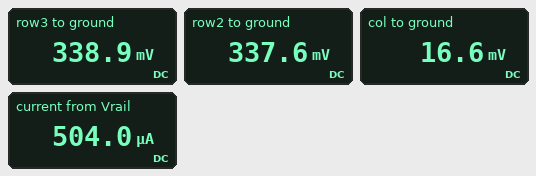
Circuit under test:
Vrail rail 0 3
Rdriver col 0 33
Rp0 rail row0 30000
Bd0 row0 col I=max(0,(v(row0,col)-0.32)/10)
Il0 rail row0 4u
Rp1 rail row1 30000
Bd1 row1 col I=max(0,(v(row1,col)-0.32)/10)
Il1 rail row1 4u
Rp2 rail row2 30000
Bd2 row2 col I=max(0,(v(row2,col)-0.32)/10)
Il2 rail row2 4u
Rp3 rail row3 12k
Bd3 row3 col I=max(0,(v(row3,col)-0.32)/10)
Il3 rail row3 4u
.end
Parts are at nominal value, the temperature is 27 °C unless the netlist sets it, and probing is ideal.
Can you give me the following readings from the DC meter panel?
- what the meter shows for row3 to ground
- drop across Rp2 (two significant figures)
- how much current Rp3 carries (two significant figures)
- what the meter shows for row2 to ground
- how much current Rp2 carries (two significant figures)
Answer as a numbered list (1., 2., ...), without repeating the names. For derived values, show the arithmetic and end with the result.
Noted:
1. 338.9 mV
2. 3 V - 337.6 mV = 2.7 V
3. (3 V - 338.9 mV) / 12 kΩ = 220 µA
4. 337.6 mV
5. (3 V - 337.6 mV) / 30 kΩ = 89 µA
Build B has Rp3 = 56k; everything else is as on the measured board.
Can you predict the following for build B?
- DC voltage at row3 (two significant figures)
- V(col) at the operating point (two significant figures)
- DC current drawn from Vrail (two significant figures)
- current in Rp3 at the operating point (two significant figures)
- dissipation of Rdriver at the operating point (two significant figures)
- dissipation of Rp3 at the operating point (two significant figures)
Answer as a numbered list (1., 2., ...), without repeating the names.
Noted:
1. 330 mV
2. 11 mV
3. 330 µA
4. 48 µA
5. 3.6 µW
6. 130 µW
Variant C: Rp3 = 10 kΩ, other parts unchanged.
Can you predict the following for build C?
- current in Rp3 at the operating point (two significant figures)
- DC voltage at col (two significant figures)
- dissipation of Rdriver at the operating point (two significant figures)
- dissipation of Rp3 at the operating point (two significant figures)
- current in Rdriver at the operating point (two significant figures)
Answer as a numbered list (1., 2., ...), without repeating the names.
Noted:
1. 270 µA
2. 18 mV
3. 9.9 µW
4. 710 µW
5. 550 µA
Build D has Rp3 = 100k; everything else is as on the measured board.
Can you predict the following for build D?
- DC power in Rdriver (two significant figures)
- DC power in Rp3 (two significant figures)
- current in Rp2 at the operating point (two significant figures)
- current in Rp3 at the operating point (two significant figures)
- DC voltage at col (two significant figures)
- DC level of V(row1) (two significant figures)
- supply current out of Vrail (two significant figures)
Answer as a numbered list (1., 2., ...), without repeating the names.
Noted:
1. 3.2 µW
2. 71 µW
3. 89 µA
4. 27 µA
5. 10 mV
6. 330 mV
7. 310 µA
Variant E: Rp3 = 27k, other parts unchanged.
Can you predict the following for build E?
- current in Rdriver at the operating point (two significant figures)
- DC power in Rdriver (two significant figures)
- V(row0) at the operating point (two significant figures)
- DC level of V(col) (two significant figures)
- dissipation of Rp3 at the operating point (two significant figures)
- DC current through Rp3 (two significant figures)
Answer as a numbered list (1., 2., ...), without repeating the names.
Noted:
1. 380 µA
2. 4.8 µW
3. 330 mV
4. 13 mV
5. 260 µW
6. 99 µA
